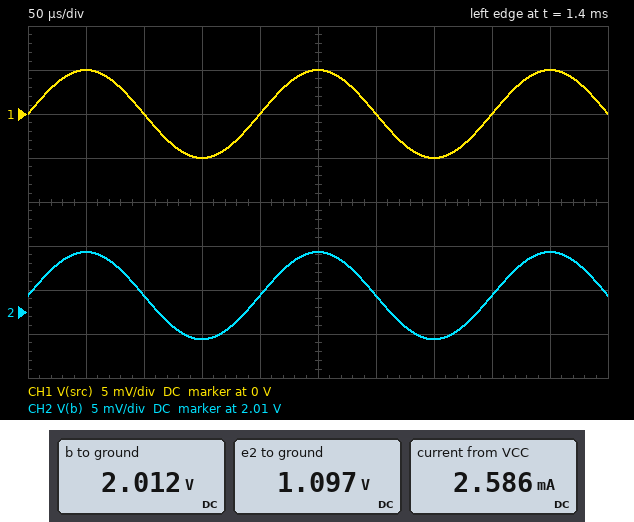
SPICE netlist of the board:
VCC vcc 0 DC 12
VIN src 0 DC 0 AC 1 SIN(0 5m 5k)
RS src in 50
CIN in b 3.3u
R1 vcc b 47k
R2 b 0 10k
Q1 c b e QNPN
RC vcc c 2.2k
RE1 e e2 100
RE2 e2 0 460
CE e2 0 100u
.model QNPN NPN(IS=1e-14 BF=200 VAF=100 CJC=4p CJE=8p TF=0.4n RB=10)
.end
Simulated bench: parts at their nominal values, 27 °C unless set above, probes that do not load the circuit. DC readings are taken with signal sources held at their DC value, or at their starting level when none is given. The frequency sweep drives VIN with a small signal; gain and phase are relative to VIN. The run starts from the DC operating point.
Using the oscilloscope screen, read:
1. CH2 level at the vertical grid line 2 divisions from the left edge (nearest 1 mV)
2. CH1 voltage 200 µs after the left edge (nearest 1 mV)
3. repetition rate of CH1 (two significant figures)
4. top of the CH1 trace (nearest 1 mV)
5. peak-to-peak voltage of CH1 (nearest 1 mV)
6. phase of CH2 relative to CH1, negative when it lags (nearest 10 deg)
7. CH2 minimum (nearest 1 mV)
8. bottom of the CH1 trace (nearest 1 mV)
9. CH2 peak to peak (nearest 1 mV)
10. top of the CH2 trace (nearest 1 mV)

2.012 V
0 V
5.0 kHz
5 mV
10 mV
0 deg
2.007 V
-5 mV
10 mV
2.017 V
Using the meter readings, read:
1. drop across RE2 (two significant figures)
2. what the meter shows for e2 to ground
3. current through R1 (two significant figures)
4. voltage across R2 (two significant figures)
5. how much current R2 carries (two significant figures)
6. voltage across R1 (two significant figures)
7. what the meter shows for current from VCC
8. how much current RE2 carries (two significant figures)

1.1 V
1.097 V
210 µA
2.0 V
200 µA
10 V
2.586 mA
2.4 mA
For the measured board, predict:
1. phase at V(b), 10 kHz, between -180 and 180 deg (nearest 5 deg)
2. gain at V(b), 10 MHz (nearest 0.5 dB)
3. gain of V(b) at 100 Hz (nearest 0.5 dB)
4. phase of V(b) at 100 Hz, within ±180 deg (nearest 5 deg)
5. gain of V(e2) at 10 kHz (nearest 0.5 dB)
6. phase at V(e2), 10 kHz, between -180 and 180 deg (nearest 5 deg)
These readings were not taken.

0 deg
-0.5 dB
0 dB
5 deg
-57.0 dB
-90 deg
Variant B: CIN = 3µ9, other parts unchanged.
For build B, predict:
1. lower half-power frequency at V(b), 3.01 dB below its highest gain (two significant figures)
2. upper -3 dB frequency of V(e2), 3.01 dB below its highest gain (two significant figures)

5.9 Hz
28 Hz
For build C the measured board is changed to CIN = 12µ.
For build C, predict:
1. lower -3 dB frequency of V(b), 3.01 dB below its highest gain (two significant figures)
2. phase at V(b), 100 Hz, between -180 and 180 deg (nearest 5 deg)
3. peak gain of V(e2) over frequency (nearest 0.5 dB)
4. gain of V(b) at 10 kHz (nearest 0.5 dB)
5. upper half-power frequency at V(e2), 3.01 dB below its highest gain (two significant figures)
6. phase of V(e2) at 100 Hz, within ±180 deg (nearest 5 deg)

1.8 Hz
0 deg
-3.0 dB
0 dB
21 Hz
-80 deg
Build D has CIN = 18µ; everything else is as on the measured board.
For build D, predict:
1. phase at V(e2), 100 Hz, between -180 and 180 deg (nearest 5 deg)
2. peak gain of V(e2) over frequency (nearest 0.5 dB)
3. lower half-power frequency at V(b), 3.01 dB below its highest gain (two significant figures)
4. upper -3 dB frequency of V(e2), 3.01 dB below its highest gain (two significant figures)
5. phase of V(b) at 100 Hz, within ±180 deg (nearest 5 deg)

-80 deg
-2.5 dB
1.2 Hz
20 Hz
0 deg
